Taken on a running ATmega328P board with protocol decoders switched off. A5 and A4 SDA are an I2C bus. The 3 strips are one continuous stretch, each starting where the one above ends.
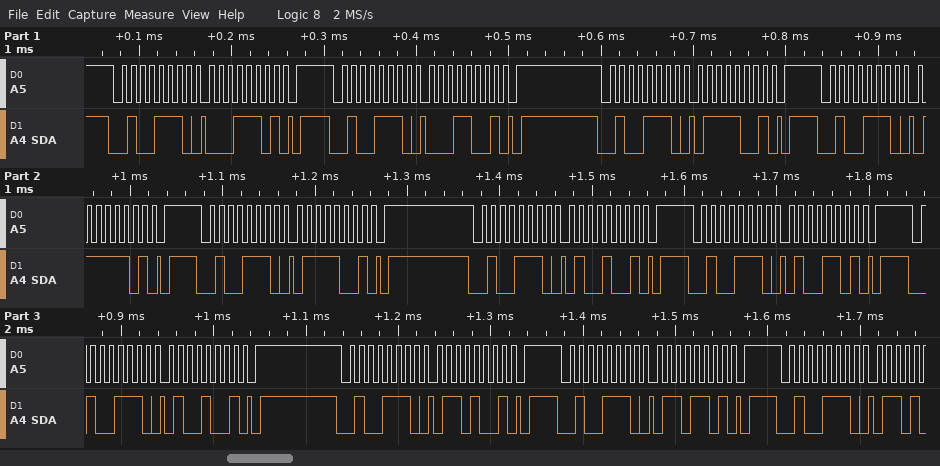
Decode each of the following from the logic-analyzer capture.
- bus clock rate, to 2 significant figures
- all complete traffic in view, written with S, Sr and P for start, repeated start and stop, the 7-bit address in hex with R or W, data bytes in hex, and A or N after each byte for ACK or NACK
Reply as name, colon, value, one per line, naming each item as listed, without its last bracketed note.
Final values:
bus clock rate, to 2 significant figures: 100 kHz
all complete traffic in view, written with S, Sr and P for start, repeated start and stop, the 7-bit address in hex with R or W, data bytes in hex, and A or N after each byte for ACK or NACK: S 27W A 1D A P S 27W A 19 A P S 27W A 79 A P S 27W A 7D A P S 27W A 79 A P S 27W A 49 A P S 27W A 4D A P S 27W A 49 A P S 27W A 69 A P S 27W A 6D A P S 27W A
